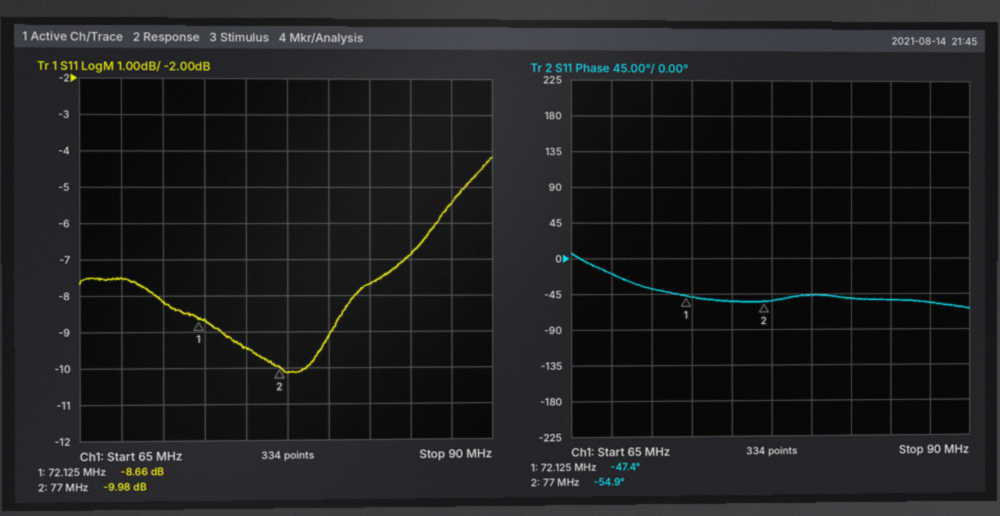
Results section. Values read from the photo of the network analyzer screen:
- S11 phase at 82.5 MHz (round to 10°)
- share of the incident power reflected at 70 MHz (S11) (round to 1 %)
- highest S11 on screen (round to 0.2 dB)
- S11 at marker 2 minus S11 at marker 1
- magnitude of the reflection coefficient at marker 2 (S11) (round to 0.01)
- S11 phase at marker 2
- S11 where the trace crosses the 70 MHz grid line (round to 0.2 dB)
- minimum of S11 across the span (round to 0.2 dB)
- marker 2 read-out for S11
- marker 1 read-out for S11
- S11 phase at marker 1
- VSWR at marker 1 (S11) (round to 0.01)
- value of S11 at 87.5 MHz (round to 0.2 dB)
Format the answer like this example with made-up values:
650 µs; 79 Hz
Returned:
-50°; 15 %; -4.2 dB; -1.32 dB; 0.32; -54.9°; -8.2 dB; -10.2 dB; -9.98 dB; -8.66 dB; -47.4°; 2.17; -5.4 dB
